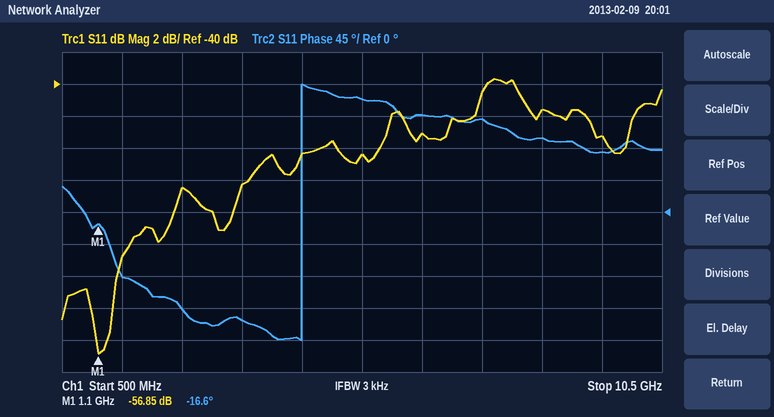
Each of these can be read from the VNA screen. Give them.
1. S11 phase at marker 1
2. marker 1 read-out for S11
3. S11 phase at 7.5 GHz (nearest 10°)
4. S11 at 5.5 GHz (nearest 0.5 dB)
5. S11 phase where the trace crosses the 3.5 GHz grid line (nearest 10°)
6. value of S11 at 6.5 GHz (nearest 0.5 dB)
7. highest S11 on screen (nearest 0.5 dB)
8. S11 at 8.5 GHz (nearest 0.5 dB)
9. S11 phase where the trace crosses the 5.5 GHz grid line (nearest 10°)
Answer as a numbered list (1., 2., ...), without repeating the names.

1. -16.6°
2. -56.85 dB
3. 130°
4. -44.5 dB
5. -150°
6. -43.0 dB
7. -39.5 dB
8. -41.5 dB
9. 160°
